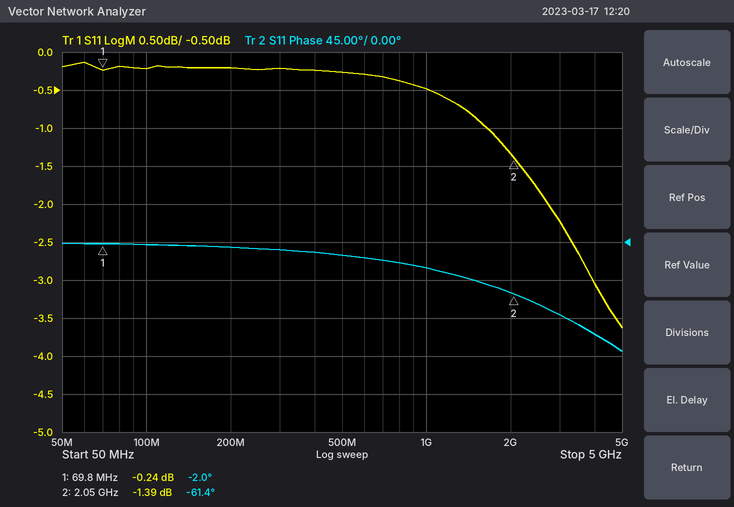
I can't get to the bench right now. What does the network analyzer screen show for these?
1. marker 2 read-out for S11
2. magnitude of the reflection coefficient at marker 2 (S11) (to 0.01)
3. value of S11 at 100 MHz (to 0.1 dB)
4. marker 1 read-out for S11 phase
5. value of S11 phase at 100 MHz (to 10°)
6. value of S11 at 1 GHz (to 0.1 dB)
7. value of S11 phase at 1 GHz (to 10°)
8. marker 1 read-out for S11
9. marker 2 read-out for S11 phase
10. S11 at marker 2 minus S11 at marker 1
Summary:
-1.39 dB
0.85
-0.2 dB
-2.0°
0°
-0.5 dB
-30°
-0.24 dB
-61.4°
-1.15 dB
